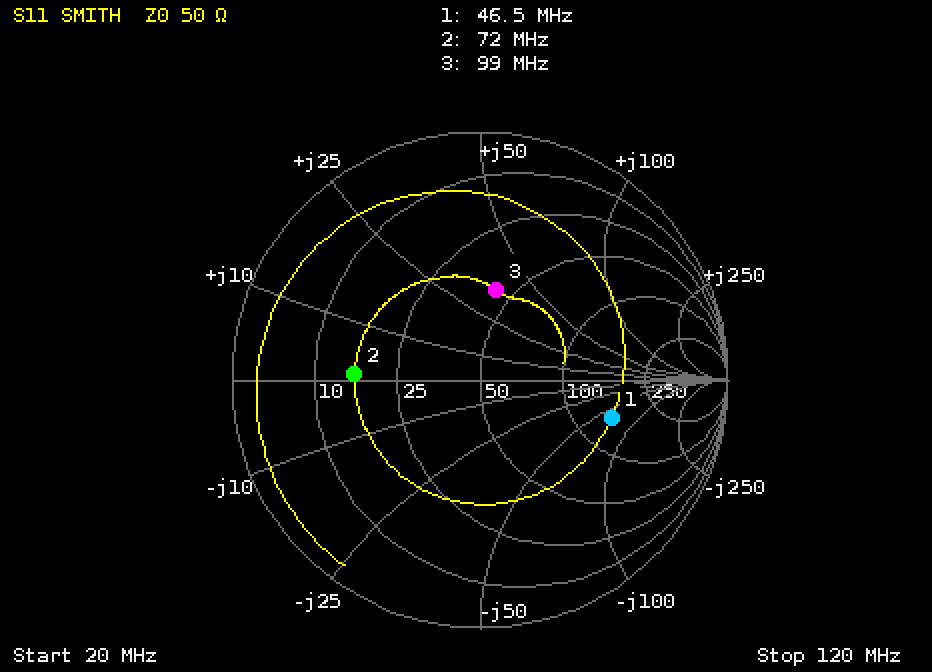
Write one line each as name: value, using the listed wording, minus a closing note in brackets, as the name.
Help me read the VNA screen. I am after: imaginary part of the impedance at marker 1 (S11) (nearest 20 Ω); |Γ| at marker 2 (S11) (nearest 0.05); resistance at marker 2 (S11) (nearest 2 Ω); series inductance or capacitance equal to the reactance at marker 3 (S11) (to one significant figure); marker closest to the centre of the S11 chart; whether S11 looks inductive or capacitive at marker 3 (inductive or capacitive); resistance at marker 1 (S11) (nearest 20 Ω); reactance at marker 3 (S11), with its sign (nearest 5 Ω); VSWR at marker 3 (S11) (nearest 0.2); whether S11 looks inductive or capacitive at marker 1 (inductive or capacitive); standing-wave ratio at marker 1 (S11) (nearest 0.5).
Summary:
imaginary part of the impedance at marker 1 (S11): -60 Ω
|Γ| at marker 2 (S11): 0.50
resistance at marker 2 (S11): 16 Ω
series inductance or capacitance equal to the reactance at marker 3 (S11): 60 nH
marker closest to the centre of the S11 chart: marker 3
whether S11 looks inductive or capacitive at marker 3: inductive
resistance at marker 1 (S11): 140 Ω
reactance at marker 3 (S11), with its sign: +35 Ω
VSWR at marker 3 (S11): 2.2
whether S11 looks inductive or capacitive at marker 1: capacitive
standing-wave ratio at marker 1 (S11): 3.5
